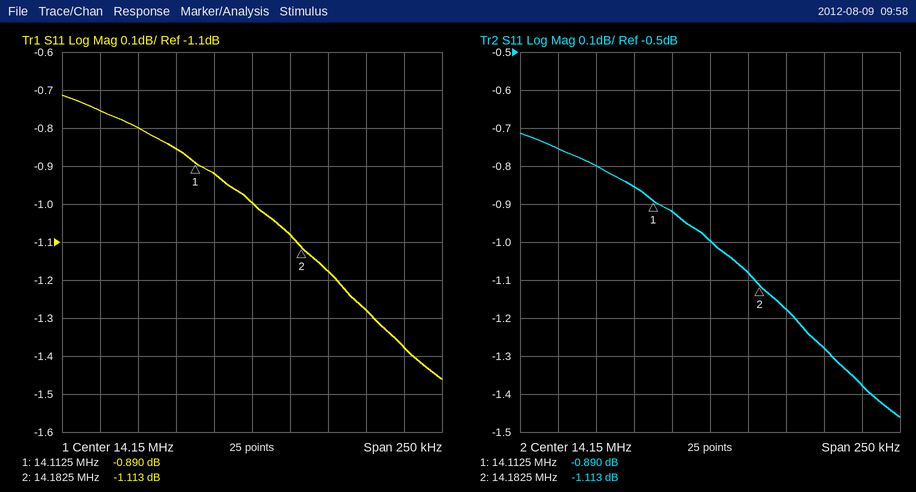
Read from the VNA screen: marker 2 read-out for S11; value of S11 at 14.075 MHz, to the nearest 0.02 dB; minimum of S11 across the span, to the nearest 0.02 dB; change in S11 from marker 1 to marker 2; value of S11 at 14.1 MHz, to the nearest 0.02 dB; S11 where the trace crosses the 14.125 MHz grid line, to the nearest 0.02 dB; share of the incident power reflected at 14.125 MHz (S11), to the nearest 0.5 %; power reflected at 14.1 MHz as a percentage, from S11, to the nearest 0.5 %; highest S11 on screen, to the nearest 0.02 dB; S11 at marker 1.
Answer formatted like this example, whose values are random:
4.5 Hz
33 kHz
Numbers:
-1.113 dB
-0.80 dB
-1.46 dB
-0.223 dB
-0.86 dB
-0.92 dB
81.0 %
82.0 %
-0.72 dB
-0.890 dB
